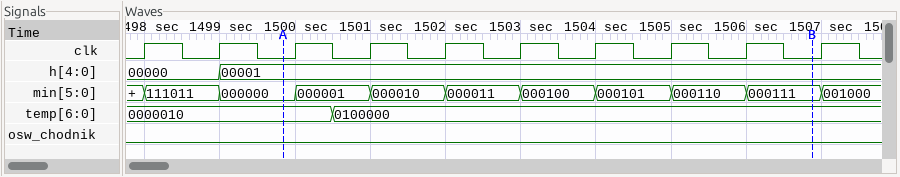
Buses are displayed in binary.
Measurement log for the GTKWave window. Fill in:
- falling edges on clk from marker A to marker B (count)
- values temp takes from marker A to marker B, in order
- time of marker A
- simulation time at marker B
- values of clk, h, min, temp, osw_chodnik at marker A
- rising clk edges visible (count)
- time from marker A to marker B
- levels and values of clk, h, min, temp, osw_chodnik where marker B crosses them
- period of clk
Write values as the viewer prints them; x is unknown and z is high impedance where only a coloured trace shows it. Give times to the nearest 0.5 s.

7
0000010, 0100000
1500 s
1507 s
clk=0, h=00001, min=000000, temp=0000010, osw_chodnik=0
10
7 s
clk=0, h=00001, min=000111, temp=0100000, osw_chodnik=0
1 s
